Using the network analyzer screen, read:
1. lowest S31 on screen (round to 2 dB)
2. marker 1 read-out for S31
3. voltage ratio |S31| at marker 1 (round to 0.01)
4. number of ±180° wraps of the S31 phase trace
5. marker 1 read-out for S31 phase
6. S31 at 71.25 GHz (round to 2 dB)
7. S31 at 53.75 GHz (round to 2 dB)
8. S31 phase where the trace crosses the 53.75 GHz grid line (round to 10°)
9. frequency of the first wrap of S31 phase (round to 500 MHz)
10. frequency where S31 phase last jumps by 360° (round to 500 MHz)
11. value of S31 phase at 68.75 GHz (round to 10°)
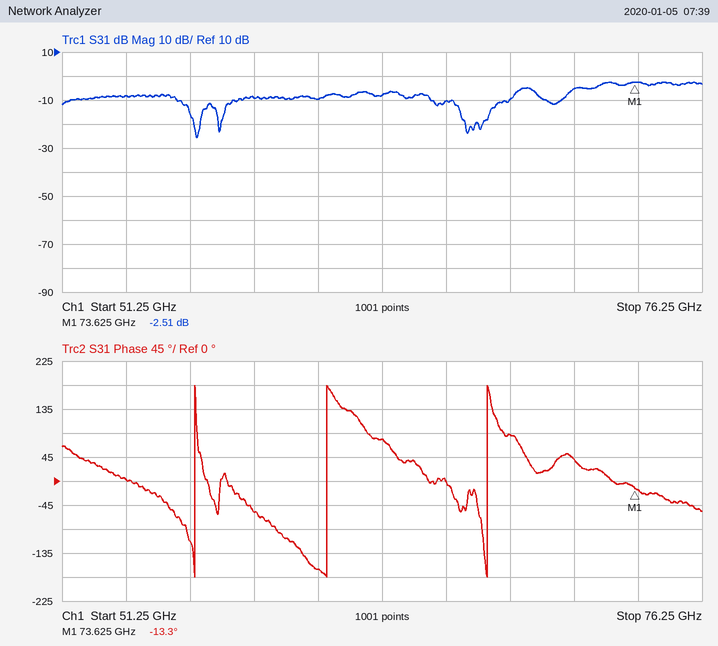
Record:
-26 dB
-2.51 dB
0.75
3
-13.3°
-6 dB
-8 dB
0°
56.5 GHz
68.0 GHz
90°
